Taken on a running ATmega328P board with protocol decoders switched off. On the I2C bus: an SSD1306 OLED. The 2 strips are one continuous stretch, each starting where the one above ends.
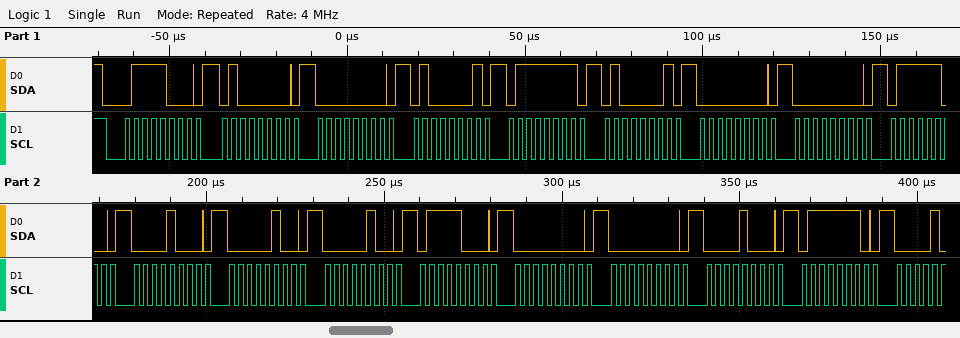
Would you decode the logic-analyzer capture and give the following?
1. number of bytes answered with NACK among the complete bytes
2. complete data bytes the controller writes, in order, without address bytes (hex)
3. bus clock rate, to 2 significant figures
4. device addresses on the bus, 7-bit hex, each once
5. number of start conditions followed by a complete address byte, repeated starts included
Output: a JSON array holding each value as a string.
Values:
["0", "40 00 41 7F 41 00 00 7C 08 04 04 78 00 00 08 7E", "400 kHz", "0x3C", "1"]
